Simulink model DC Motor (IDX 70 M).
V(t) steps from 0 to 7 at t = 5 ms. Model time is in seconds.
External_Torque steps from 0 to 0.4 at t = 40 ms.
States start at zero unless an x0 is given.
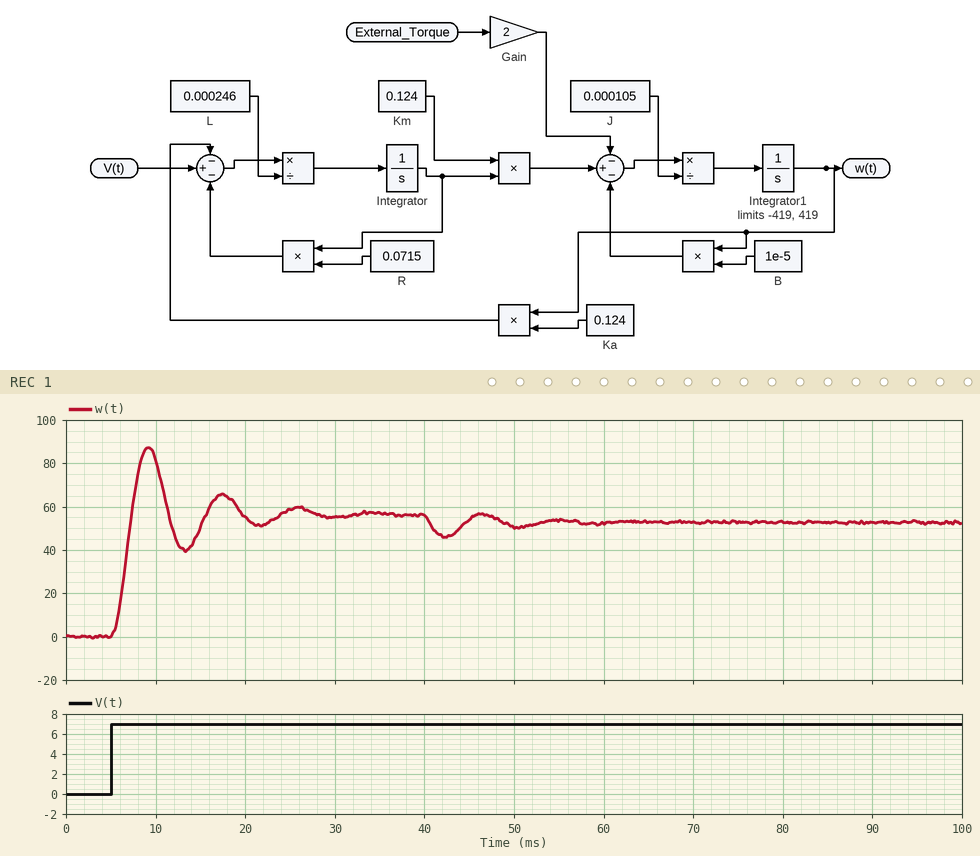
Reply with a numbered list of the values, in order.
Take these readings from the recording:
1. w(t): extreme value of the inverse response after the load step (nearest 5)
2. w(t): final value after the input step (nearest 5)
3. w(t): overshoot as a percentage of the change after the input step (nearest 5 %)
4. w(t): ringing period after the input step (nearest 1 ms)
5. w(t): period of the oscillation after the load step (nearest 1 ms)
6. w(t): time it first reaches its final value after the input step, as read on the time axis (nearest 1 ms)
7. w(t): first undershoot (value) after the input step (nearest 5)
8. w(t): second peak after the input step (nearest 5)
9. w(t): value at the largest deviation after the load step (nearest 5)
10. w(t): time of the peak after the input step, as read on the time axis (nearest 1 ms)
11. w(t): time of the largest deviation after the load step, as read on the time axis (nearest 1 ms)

1. 55
2. 55
3. 55 %
4. 8 ms
5. 8 ms
6. 7 ms
7. 40
8. 65
9. 45
10. 9 ms
11. 42 ms
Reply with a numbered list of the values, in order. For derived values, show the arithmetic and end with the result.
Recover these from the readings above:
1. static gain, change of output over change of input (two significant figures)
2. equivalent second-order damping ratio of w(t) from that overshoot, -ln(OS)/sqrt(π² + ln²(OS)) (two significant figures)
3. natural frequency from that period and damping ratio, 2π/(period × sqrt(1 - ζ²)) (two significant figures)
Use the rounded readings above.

1. (55 - 0) / (7 - 0) = 7.9
2. ln(0.55) = -0.598; 0.598 / sqrt(9.870 + 0.357) = 0.19
3. 2π / (8 × sqrt(1 - 0.19²)) = 0.80 rad/ms
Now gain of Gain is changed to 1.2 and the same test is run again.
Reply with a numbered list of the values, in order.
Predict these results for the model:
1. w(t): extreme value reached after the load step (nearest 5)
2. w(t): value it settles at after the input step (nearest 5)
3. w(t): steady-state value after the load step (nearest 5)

1. 50
2. 55
3. 55
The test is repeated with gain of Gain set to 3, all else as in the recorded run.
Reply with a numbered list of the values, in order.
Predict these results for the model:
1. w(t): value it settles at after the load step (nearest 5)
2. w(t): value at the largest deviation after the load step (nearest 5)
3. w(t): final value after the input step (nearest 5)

1. 50
2. 40
3. 55
